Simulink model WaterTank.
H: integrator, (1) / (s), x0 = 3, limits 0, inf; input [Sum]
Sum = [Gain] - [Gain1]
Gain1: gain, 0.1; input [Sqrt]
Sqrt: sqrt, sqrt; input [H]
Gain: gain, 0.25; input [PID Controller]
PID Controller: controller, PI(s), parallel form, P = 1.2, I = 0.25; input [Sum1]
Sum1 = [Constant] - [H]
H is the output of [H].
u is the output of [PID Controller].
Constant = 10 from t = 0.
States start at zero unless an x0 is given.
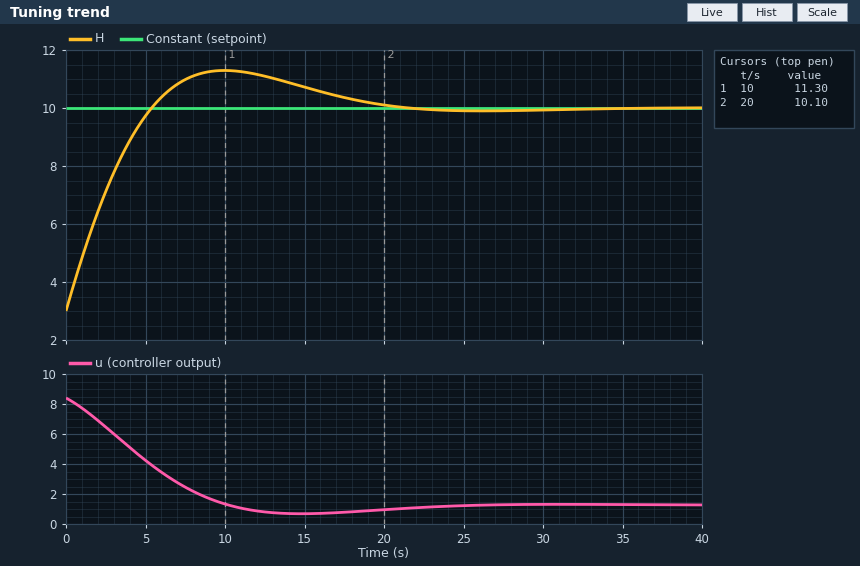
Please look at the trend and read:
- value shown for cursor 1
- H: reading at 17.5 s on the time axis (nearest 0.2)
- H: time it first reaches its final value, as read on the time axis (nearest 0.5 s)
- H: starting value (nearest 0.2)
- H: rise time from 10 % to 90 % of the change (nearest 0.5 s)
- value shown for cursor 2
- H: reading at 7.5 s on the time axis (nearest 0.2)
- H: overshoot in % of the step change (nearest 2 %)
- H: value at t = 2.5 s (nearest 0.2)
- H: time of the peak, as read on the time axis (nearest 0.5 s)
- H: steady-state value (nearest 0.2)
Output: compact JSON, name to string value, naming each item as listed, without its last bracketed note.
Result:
{"value shown for cursor 1": "11.30", "H: reading at 17.5 s on the time axis": "10.4", "H: time it first reaches its final value, as read on the time axis": "5.5 s", "H: starting value": "3.0", "H: rise time from 10 % to 90 % of the change": "4.0 s", "value shown for cursor 2": "10.10", "H: reading at 7.5 s on the time axis": "11.0", "H: overshoot in % of the step change": "18 %", "H: value at t = 2.5 s": "7.2", "H: time of the peak, as read on the time axis": "10.0 s", "H: steady-state value": "10.0"}
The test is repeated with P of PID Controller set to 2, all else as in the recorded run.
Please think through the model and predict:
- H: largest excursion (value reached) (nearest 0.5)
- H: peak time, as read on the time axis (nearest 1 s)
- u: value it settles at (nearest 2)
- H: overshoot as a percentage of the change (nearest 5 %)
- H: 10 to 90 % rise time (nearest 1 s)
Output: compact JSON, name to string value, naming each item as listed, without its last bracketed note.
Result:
{"H: largest excursion (value reached)": "10.5", "H: peak time, as read on the time axis": "9 s", "u: value it settles at": "2", "H: overshoot as a percentage of the change": "10 %", "H: 10 to 90 % rise time": "3 s"}
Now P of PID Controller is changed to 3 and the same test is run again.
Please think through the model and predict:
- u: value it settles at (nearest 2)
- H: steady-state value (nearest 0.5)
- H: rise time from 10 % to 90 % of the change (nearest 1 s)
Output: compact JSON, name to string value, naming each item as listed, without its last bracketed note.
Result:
{"u: value it settles at": "2", "H: steady-state value": "10.0", "H: rise time from 10 % to 90 % of the change": "3 s"}
